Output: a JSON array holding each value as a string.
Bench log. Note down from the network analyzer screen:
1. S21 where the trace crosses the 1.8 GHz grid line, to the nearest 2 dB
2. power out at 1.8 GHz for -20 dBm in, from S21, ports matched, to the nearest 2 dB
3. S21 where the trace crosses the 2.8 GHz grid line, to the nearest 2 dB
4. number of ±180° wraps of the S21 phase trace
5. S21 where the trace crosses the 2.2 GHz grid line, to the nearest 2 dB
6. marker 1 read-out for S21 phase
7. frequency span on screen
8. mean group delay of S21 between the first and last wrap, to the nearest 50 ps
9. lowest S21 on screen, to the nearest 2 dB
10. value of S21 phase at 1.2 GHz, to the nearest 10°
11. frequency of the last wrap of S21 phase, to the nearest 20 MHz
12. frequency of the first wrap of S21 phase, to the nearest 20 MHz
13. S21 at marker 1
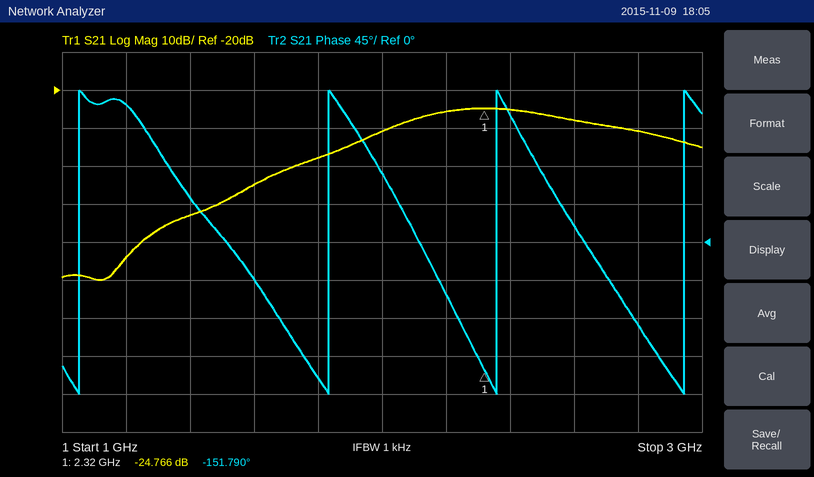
["-38 dB", "-58 dBm", "-30 dB", "4", "-26 dB", "-151.790°", "2 GHz", "1.60 ns", "-70 dB", "160°", "2.94 GHz", "1.06 GHz", "-24.766 dB"]
